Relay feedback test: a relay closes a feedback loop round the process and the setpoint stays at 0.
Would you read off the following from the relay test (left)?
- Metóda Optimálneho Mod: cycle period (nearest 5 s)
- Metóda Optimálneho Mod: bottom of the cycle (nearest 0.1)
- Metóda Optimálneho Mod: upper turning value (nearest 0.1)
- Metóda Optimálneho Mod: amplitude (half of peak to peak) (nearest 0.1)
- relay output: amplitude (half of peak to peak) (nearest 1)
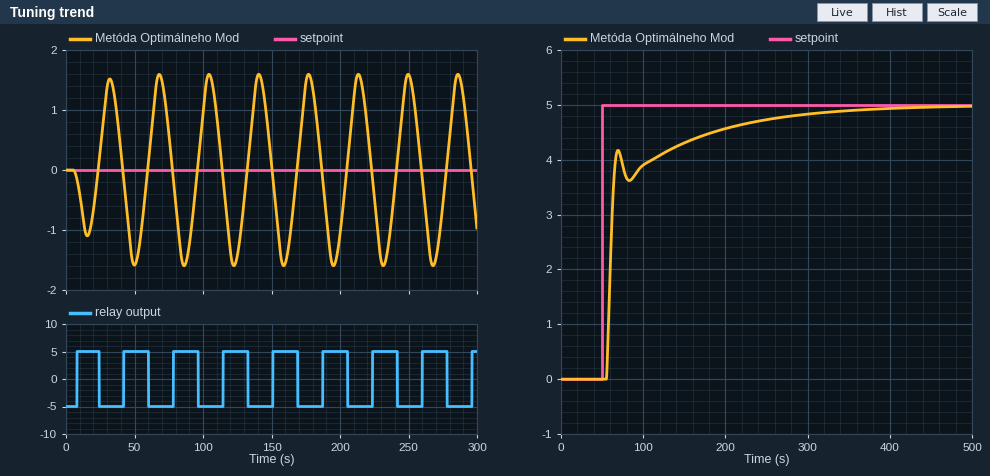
35 s
-1.6
1.6
1.6
5
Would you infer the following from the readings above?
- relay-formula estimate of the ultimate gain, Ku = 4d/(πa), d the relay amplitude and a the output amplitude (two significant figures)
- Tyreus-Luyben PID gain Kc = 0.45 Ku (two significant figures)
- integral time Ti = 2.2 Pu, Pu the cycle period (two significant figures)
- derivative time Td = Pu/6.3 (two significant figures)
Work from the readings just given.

4.0
1.8
77 s
5.6 s
